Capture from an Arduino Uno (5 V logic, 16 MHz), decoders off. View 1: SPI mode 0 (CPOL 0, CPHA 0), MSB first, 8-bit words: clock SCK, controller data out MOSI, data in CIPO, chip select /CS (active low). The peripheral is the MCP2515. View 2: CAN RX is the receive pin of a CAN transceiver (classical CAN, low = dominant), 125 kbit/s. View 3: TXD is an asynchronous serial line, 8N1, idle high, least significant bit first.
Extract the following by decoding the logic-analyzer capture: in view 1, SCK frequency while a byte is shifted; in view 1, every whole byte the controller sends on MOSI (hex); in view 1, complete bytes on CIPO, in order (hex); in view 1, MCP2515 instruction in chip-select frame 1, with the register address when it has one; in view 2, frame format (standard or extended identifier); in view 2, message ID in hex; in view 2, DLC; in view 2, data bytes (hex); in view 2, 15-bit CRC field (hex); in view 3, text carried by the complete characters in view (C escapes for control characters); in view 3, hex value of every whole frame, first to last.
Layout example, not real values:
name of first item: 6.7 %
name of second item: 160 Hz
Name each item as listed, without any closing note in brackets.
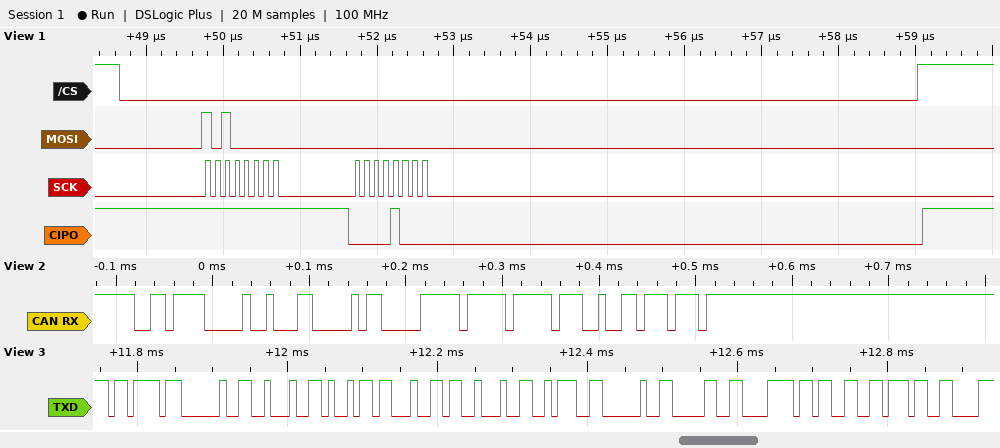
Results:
in view 1, SCK frequency while a byte is shifted: 8 MHz
in view 1, every whole byte the controller sends on MOSI: 0xA0 0x00
in view 1, complete bytes on CIPO, in order: 0xFF 0x08
in view 1, MCP2515 instruction in chip-select frame 1, with the register address when it has one: READ STATUS
in view 2, frame format: standard
in view 2, message ID in hex: 0x378
in view 2, DLC: 4
in view 2, data bytes: 60 60 FF FF
in view 2, 15-bit CRC field: 0x49BB
in view 3, text carried by the complete characters in view: "{ \"id\": 0x37"
in view 3, hex value of every whole frame, first to last: 7B 20 22 69 64 22 3A 20 30 78 33 37
